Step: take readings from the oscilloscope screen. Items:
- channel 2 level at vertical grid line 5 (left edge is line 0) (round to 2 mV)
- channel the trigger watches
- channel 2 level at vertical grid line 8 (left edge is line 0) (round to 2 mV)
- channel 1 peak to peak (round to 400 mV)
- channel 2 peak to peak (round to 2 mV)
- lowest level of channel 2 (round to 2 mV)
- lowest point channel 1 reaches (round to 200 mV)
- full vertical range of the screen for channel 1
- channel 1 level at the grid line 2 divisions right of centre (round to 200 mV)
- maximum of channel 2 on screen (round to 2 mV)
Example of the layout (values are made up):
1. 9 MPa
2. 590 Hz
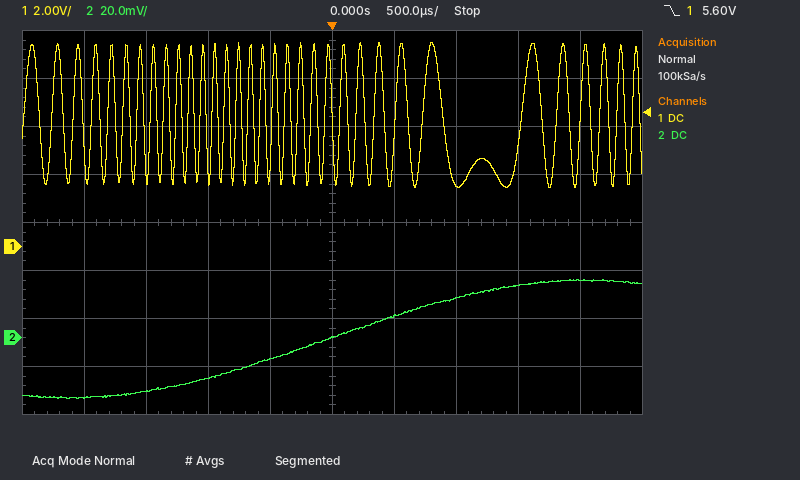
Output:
1. 0 mV
2. channel 1
3. 22 mV
4. 6.0 V
5. 50 mV
6. -26 mV
7. 2.4 V
8. 16 V
9. 2.6 V
10. 24 mV
